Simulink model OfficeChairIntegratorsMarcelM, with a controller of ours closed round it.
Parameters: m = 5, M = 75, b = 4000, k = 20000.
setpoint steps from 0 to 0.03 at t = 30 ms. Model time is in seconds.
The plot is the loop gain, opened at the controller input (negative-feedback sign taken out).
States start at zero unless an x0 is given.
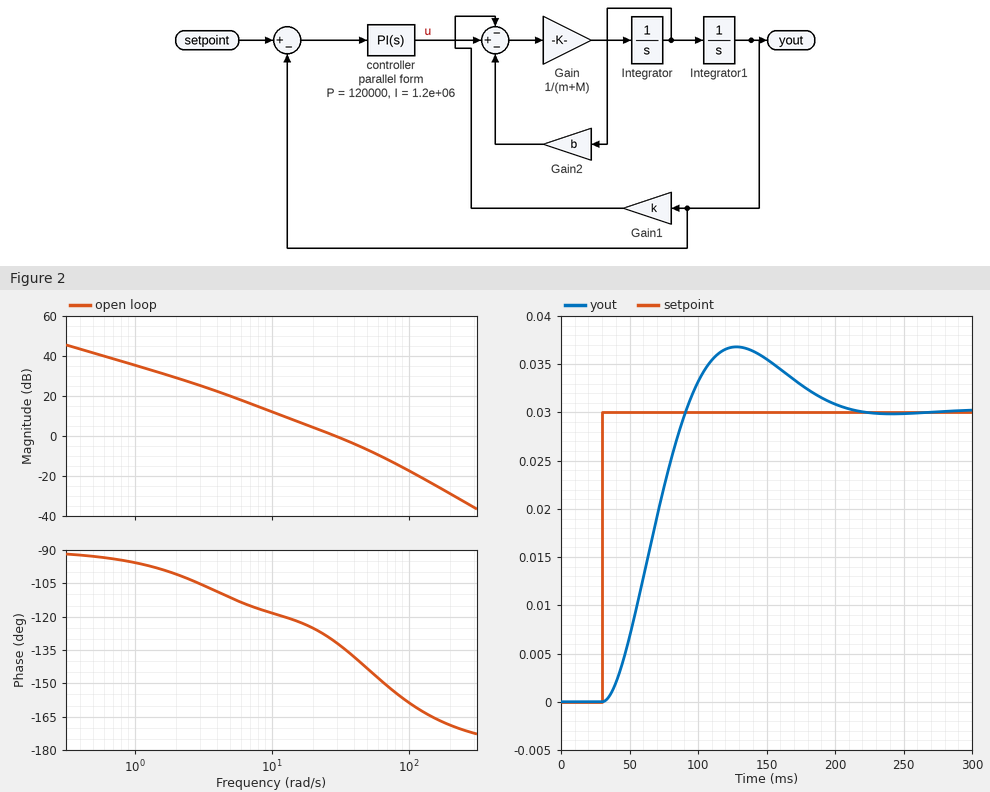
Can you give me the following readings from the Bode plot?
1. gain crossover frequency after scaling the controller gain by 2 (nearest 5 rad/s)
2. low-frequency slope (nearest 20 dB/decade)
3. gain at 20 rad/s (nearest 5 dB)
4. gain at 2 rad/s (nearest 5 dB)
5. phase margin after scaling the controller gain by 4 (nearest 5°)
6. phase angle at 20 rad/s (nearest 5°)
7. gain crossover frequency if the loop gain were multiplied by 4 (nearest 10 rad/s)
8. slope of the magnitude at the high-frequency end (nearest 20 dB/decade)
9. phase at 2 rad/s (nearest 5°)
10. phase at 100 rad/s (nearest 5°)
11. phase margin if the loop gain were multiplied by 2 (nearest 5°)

45 rad/s
-20 dB/decade
5 dB
30 dB
30°
-125°
70 rad/s
-40 dB/decade
-100°
-160°
40°
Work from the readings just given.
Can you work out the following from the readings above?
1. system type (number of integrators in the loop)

1
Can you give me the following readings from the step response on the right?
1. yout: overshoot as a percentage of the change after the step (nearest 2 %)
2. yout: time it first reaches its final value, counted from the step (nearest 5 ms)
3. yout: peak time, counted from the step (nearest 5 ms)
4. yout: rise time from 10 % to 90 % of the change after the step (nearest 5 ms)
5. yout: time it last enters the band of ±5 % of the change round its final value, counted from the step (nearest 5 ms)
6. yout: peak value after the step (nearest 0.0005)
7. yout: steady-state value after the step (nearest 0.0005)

22 %
60 ms
100 ms
40 ms
160 ms
0.0370
0.0300
